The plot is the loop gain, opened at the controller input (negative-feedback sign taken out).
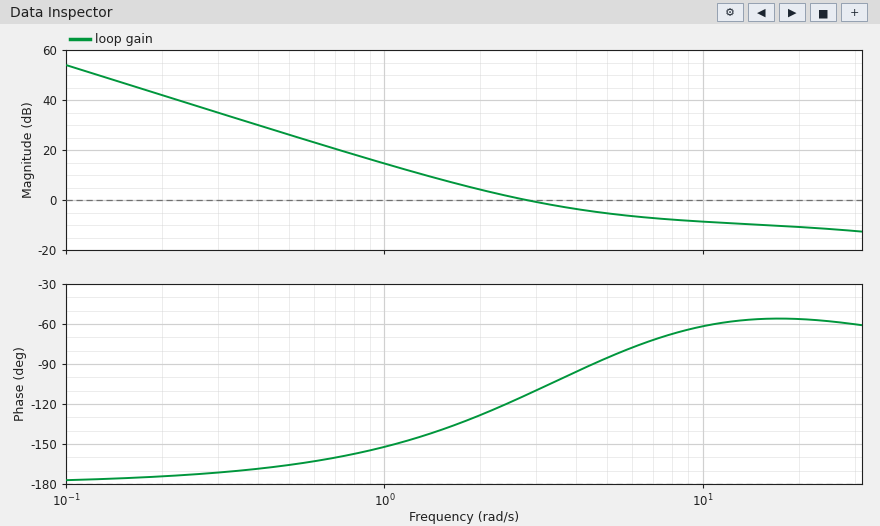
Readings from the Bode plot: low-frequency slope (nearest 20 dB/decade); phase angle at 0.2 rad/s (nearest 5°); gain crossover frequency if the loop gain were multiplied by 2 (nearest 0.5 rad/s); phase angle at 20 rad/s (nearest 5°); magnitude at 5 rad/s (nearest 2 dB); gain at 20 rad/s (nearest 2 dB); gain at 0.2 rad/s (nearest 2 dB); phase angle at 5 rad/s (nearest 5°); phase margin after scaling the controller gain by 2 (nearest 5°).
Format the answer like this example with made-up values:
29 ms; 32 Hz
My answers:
-40 dB/decade; -175°; 5.5 rad/s; -55°; -6 dB; -10 dB; 42 dB; -85°; 100°
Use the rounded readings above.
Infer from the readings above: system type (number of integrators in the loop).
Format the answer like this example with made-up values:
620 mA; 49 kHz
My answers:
2
